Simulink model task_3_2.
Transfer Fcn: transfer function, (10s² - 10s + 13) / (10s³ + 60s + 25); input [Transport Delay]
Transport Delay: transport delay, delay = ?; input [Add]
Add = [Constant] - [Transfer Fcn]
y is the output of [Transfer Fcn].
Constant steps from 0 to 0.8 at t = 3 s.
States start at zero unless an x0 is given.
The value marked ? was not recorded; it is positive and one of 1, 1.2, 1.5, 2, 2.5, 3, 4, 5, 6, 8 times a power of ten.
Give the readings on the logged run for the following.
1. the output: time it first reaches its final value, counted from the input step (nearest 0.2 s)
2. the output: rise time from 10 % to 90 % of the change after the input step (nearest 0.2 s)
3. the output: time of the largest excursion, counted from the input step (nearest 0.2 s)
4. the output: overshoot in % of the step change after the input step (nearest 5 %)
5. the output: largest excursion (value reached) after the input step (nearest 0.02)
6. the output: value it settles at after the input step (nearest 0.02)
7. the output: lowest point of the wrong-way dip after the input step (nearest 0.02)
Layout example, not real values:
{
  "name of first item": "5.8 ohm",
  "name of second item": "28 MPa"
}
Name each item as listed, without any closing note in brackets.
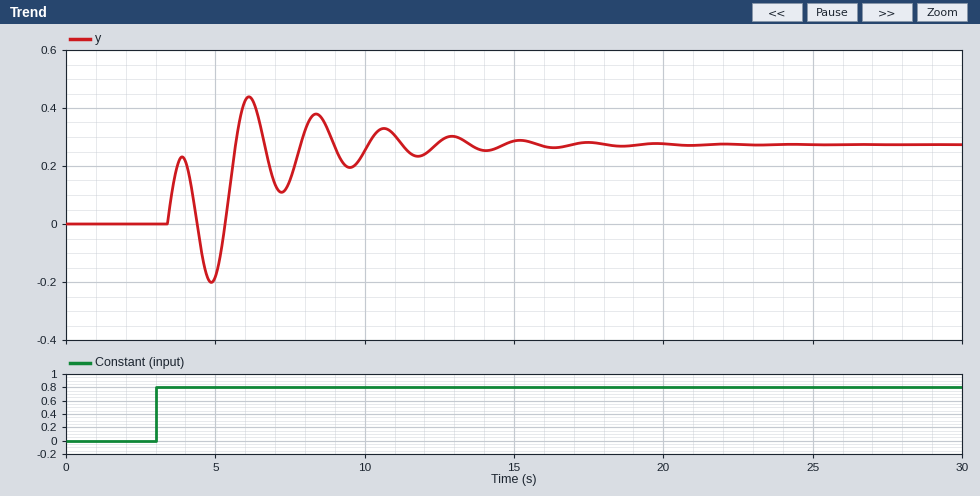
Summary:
{
  "the output: time it first reaches its final value, counted from the input step": "2.6 s",
  "the output: rise time from 10 % to 90 % of the change after the input step": "2.2 s",
  "the output: time of the largest excursion, counted from the input step": "3.2 s",
  "the output: overshoot in % of the step change after the input step": "60 %",
  "the output: largest excursion (value reached) after the input step": "0.44",
  "the output: value it settles at after the input step": "0.28",
  "the output: lowest point of the wrong-way dip after the input step": "-0.20"
}
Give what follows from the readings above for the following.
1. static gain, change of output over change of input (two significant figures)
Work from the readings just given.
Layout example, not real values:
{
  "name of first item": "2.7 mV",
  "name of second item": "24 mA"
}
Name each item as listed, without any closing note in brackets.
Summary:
{
  "static gain, change of output over change of input": "0.35"
}
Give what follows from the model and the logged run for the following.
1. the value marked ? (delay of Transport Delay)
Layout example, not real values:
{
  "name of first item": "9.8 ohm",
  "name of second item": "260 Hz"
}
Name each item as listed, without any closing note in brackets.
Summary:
{
  "the value marked ?": "0.4"
}
